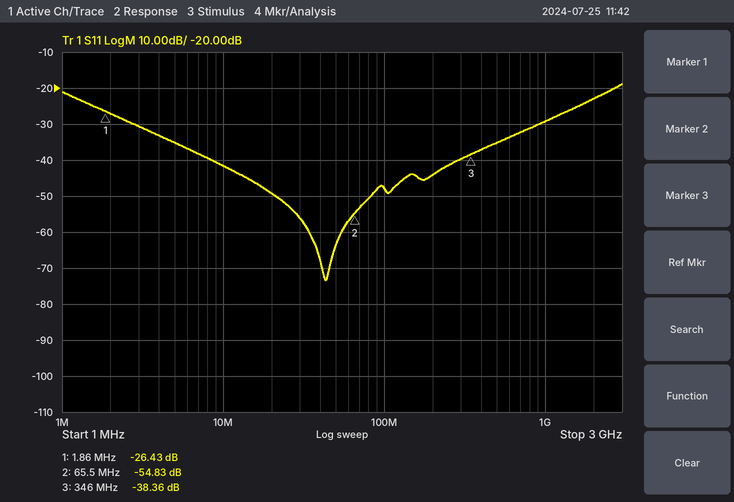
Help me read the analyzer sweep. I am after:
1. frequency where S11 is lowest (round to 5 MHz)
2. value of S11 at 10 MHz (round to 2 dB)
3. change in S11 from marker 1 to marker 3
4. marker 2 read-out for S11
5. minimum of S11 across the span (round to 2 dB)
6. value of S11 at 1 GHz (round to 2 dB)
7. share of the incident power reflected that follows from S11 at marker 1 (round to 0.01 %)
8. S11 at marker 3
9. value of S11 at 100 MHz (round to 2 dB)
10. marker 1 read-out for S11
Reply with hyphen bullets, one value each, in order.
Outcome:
- 45 MHz
- -42 dB
- -11.93 dB
- -54.83 dB
- -74 dB
- -30 dB
- 0.23 %
- -38.36 dB
- -48 dB
- -26.43 dB
